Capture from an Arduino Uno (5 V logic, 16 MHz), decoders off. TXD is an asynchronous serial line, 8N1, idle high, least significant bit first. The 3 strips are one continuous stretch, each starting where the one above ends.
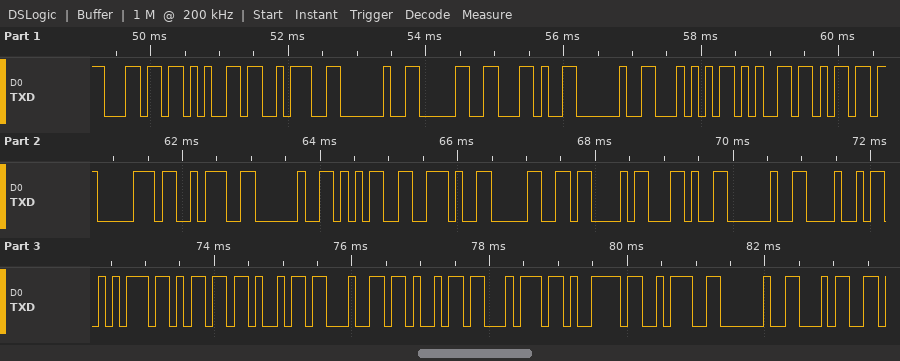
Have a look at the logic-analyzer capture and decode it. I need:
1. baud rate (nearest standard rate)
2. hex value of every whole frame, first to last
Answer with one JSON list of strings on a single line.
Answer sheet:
["9600 baud", "6C 65 3A 20 30 2C 20 54 65 6D 70 3A 20 35 2E 30 43 2C 20 48 75 6D 69 64 69 74 79 3A 20 34"]
